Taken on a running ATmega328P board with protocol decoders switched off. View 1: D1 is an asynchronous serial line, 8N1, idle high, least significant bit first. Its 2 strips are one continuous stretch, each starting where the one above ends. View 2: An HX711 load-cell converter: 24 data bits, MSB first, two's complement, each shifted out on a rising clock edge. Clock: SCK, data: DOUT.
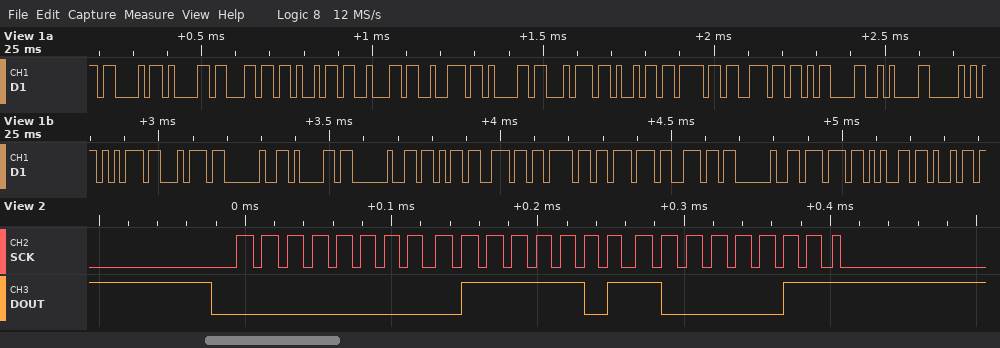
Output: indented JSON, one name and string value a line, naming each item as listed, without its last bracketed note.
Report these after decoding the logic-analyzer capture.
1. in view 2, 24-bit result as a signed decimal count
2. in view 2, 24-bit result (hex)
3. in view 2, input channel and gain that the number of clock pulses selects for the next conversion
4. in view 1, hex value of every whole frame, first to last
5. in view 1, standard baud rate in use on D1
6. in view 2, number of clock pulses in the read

{
  "in view 2, 24-bit result as a signed decimal count": "32131",
  "in view 2, 24-bit result": "0x007D83",
  "in view 2, input channel and gain that the number of clock pulses selects for the next conversion": "channel A, gain 128",
  "in view 1, hex value of every whole frame, first to last": "43 61 6C 69 62 72 61 74 69 6F 6E 0D 0A 50 75 74 20 61 20 6B 6E 6F 77 6E 20 77 65 69",
  "in view 1, standard baud rate in use on D1": "57600 baud",
  "in view 2, number of clock pulses in the read": "25"
}
